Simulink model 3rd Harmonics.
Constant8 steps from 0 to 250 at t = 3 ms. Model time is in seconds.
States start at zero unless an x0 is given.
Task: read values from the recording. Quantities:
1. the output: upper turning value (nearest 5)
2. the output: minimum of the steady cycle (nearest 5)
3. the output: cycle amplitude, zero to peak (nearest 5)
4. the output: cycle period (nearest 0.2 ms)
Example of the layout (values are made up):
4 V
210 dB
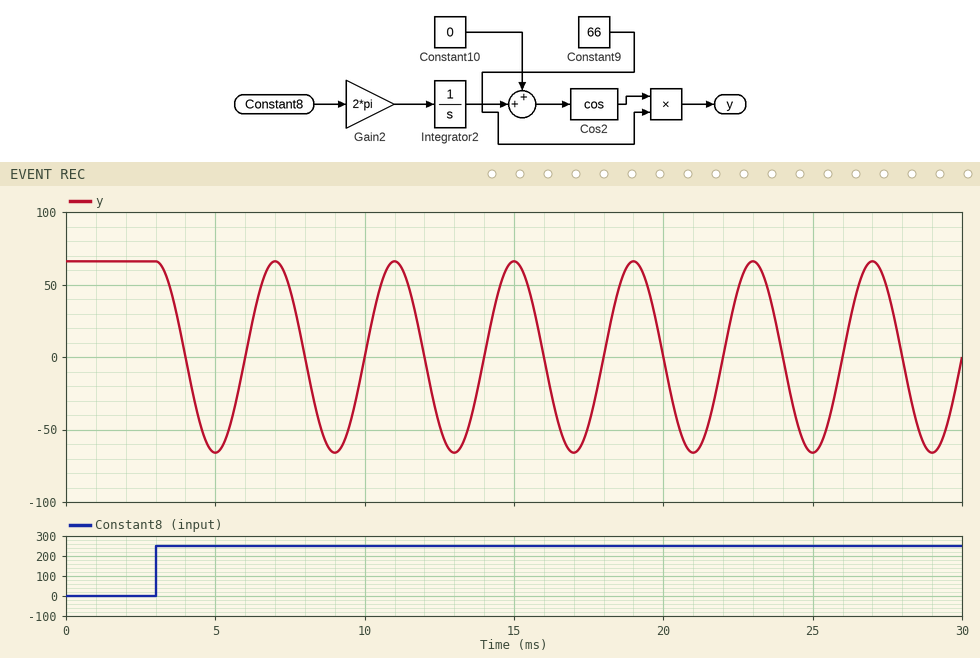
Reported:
65
-65
65
4.0 ms
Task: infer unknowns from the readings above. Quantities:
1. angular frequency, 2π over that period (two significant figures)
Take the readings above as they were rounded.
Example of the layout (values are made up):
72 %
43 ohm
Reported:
1.6 rad/ms
